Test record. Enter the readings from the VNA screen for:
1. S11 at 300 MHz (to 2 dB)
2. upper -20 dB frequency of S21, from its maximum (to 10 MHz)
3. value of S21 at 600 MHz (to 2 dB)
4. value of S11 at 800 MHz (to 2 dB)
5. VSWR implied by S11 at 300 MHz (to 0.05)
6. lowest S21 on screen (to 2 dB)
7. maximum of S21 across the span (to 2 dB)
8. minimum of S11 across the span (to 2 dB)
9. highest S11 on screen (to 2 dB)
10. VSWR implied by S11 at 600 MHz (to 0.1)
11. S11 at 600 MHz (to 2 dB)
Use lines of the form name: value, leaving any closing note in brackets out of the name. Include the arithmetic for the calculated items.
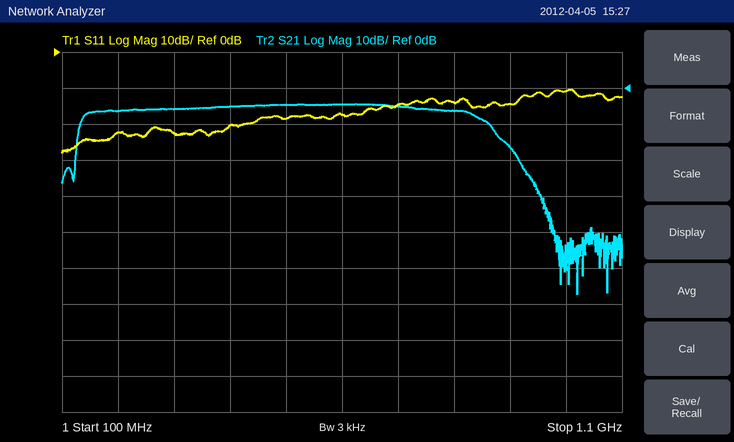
S11 at 300 MHz: -22 dB
upper -20 dB frequency of S21, from its maximum: 930 MHz
value of S21 at 600 MHz: -4 dB
value of S11 at 800 MHz: -14 dB
VSWR implied by S11 at 300 MHz: |Γ| = 10^(-22/20) = 0.0794; VSWR = (1 + 0.0794)/(1 − 0.0794) ≈ 1.17, so 1.15 to the nearest 0.05
lowest S21 on screen: -58 dB
maximum of S21 across the span: -4 dB
minimum of S11 across the span: -28 dB
highest S11 on screen: -10 dB
VSWR implied by S11 at 600 MHz: |Γ| = 10^(-18/20) = 0.1259; VSWR = (1 + 0.1259)/(1 − 0.1259) ≈ 1.3
S11 at 600 MHz: -18 dB
